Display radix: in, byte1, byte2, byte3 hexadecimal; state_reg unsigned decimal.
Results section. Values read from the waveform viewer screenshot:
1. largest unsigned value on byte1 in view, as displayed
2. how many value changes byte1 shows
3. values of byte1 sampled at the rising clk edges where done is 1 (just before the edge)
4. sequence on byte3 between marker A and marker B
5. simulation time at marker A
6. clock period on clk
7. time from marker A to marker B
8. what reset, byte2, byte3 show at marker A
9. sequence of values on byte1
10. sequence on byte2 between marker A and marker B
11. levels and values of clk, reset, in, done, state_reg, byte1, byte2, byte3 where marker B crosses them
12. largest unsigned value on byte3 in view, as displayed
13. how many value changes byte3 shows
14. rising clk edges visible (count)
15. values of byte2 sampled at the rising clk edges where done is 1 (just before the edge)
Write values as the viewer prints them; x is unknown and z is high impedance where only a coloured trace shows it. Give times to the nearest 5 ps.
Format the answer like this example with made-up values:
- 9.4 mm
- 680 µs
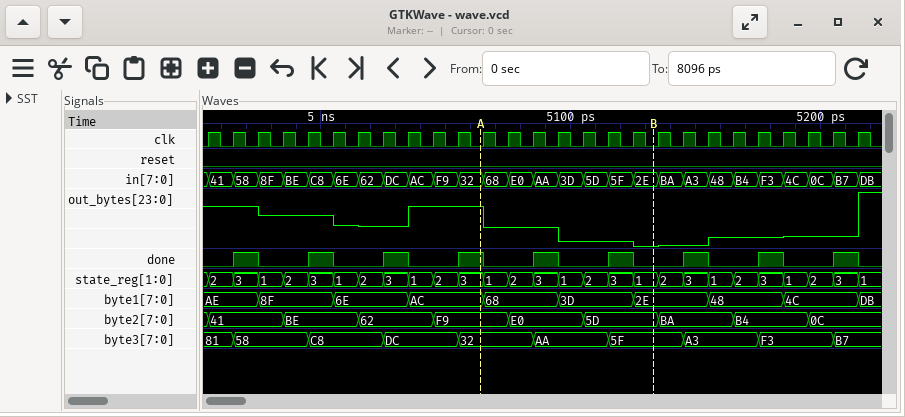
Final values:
- DB
- 9
- AE, 8F, 6E, AC, 68, 3D, 2E, 48, 4C
- 32, AA, 5F
- 5065 ps
- 10 ps
- 70 ps
- reset=0, byte2=F9, byte3=32
- AE, 8F, 6E, AC, 68, 3D, 2E, 48, 4C, DB
- F9, E0, 5D
- clk=0, reset=0, in=2E, done=0, state_reg=1, byte1=2E, byte2=5D, byte3=5F
- F3
- 9
- 27
- 41, BE, 62, F9, E0, 5D, BA, B4, 0C
